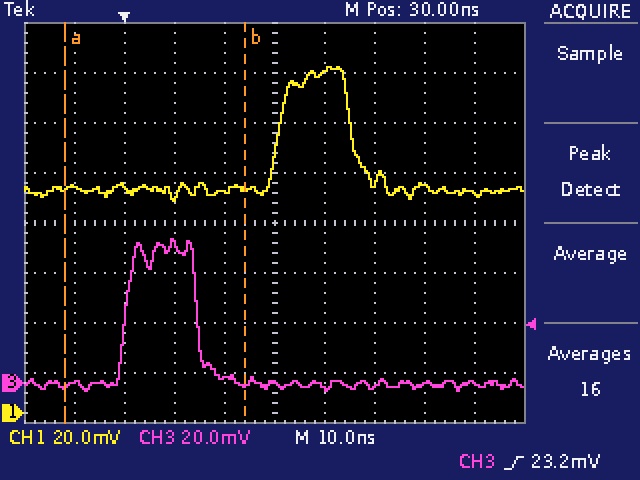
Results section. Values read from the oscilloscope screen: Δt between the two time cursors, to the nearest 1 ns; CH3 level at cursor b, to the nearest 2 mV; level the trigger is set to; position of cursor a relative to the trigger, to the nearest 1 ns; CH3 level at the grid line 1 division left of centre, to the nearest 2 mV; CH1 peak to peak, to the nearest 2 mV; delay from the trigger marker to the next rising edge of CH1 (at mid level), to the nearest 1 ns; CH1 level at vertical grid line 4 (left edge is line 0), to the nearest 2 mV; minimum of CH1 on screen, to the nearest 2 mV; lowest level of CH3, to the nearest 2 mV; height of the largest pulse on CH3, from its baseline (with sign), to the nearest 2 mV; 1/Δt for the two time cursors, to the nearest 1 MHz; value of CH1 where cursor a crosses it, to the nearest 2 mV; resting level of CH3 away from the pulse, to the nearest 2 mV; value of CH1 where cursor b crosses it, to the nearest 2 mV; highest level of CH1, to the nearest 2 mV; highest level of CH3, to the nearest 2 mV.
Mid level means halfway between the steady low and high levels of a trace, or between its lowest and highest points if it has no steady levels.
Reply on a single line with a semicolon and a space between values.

36 ns; 0 mV; 23.2 mV; -12 ns; 2 mV; 54 mV; 31 ns; 88 mV; 84 mV; -4 mV; +58 mV; 28 MHz; 90 mV; 0 mV; 90 mV; 138 mV; 58 mV
